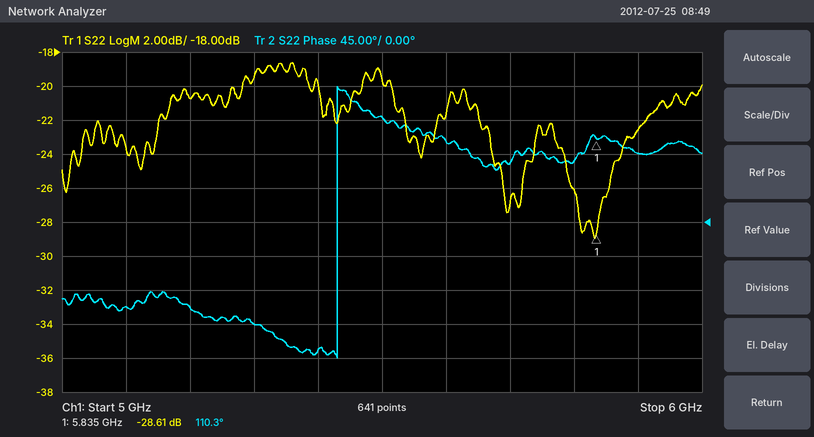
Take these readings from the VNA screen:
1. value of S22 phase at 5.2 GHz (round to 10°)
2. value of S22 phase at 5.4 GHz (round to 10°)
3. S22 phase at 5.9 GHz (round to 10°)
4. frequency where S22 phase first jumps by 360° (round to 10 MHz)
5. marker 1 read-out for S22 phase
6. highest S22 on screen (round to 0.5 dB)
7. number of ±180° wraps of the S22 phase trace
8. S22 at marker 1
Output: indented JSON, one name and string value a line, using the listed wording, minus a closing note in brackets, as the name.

{
  "value of S22 phase at 5.2 GHz": "-110°",
  "value of S22 phase at 5.4 GHz": "-170°",
  "S22 phase at 5.9 GHz": "90°",
  "frequency where S22 phase first jumps by 360°": "5.43 GHz",
  "marker 1 read-out for S22 phase": "110.3°",
  "highest S22 on screen": "-18.5 dB",
  "number of ±180° wraps of the S22 phase trace": "1",
  "S22 at marker 1": "-28.61 dB"
}
